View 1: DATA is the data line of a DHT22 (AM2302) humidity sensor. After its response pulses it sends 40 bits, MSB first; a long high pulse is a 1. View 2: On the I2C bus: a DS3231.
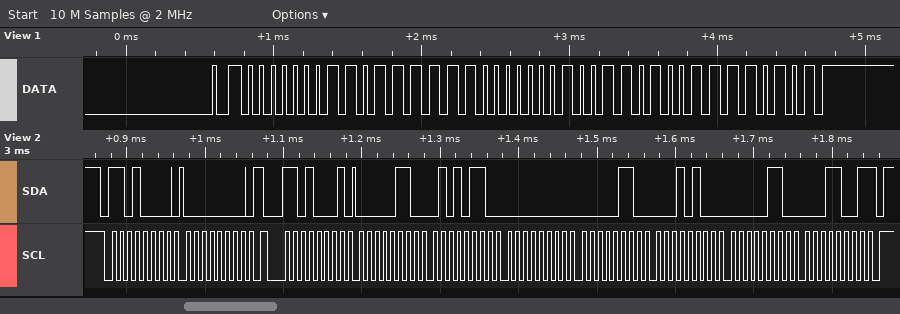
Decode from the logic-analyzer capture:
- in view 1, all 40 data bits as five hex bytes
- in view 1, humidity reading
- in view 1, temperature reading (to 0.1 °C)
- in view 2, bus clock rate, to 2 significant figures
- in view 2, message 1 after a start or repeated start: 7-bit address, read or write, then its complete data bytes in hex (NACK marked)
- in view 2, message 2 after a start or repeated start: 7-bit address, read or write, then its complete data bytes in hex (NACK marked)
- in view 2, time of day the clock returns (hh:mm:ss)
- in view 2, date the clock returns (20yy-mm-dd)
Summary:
01 BF 01 34 F5
44.7 %
30.8 °C
100 kHz
0x68 write: 00
0x68 read: 06 56 00 06 14 06 19 NACK
00:56:06
2019-06-14
